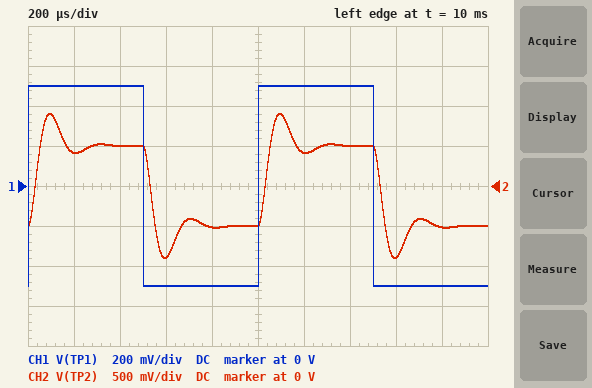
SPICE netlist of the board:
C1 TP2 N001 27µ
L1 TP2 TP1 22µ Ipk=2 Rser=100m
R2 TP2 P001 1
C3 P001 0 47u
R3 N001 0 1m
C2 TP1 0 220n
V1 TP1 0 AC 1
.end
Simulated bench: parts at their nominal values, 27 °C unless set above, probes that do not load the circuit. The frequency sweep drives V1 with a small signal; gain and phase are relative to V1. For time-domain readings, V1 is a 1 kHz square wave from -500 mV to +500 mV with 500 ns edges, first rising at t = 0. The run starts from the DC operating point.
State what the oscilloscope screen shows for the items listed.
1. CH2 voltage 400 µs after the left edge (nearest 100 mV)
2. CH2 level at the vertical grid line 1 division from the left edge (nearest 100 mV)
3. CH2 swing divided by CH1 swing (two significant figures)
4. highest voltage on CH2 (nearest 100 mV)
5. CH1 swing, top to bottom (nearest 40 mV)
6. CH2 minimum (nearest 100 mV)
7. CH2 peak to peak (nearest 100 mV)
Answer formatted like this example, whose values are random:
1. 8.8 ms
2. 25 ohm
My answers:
1. 500 mV
2. 400 mV
3. 1.8
4. 900 mV
5. 1.00 V
6. -900 mV
7. 1.8 V
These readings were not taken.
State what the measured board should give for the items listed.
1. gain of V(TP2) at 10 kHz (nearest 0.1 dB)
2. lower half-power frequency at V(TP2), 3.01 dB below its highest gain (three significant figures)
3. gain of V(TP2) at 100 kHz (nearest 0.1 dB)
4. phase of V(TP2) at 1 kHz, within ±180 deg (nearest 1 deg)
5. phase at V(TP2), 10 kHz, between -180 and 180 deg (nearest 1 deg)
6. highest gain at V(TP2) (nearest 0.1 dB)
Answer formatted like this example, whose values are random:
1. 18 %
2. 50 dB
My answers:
1. -6.9 dB
2. 1.88 kHz
3. -47.4 dB
4. -3 deg
5. -139 deg
6. 4.5 dB
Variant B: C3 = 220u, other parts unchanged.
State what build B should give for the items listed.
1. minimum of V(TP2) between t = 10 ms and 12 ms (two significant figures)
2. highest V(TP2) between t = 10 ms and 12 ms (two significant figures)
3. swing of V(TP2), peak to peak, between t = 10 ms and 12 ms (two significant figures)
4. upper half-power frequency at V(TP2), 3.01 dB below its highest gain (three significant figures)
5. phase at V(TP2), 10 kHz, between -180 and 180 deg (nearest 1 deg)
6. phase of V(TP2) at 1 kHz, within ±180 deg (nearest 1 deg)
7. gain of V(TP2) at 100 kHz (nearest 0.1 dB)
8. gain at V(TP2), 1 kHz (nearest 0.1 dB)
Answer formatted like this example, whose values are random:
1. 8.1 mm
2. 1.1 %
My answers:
1. -660 mV
2. 660 mV
3. 1.3 V
4. 7.61 kHz
5. -131 deg
6. -9 deg
7. -47.4 dB
8. 0.1 dB
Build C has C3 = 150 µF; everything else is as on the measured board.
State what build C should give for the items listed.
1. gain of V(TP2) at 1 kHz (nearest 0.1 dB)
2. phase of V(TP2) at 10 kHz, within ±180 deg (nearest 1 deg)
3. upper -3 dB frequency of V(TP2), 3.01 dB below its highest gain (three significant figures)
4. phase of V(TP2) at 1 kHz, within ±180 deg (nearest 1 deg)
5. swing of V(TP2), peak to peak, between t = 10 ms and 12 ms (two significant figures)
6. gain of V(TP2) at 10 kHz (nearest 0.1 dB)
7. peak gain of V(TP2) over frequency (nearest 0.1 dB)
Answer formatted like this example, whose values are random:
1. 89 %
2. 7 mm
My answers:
1. 0.3 dB
2. -132 deg
3. 7.39 kHz
4. -8 deg
5. 1.4 V
6. -6.4 dB
7. 1.5 dB
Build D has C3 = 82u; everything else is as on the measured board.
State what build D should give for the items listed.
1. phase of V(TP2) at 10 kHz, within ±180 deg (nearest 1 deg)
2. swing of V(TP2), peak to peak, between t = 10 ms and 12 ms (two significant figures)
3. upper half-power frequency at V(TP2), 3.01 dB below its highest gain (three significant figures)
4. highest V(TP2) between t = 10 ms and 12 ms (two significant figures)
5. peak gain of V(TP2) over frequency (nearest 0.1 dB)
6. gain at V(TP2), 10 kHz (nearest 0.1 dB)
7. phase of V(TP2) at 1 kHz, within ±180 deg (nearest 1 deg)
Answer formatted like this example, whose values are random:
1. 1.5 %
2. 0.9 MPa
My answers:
1. -135 deg
2. 1.6 V
3. 6.82 kHz
4. 790 mV
5. 2.6 dB
6. -6.6 dB
7. -5 deg
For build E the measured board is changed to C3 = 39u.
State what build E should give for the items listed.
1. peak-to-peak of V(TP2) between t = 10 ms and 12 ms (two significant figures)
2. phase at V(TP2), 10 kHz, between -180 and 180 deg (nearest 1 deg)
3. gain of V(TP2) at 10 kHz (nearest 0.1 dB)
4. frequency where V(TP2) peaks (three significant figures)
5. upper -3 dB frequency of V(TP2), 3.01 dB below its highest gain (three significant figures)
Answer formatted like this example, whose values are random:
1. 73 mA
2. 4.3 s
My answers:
1. 1.9 V
2. -141 deg
3. -7.0 dB
4. 4.45 kHz
5. 6.12 kHz
